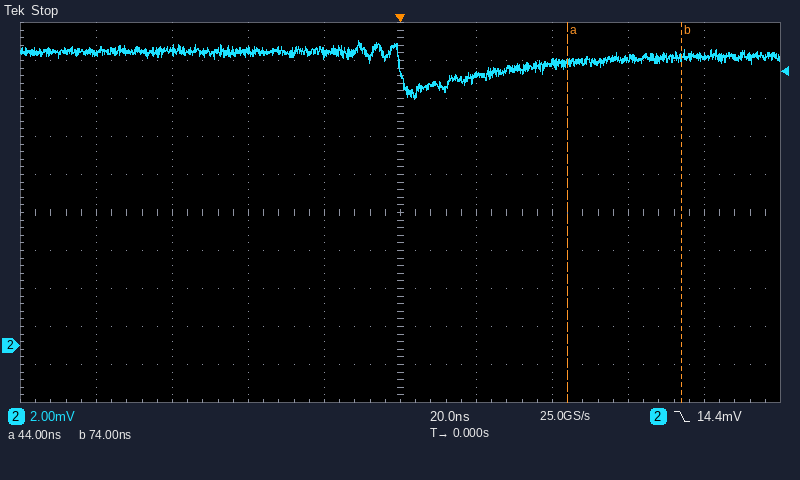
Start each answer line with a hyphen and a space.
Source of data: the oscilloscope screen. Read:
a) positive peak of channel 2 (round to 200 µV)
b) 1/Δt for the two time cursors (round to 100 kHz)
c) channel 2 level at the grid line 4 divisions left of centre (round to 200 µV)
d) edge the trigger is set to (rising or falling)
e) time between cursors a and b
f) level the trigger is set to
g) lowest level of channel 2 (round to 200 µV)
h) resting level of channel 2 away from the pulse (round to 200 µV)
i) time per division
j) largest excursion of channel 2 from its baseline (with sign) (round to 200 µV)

- 16.0 mV
- 33.3 MHz
- 15.4 mV
- falling
- 30 ns
- 14.4 mV
- 13.0 mV
- 15.4 mV
- 20 ns
- -2.4 mV
